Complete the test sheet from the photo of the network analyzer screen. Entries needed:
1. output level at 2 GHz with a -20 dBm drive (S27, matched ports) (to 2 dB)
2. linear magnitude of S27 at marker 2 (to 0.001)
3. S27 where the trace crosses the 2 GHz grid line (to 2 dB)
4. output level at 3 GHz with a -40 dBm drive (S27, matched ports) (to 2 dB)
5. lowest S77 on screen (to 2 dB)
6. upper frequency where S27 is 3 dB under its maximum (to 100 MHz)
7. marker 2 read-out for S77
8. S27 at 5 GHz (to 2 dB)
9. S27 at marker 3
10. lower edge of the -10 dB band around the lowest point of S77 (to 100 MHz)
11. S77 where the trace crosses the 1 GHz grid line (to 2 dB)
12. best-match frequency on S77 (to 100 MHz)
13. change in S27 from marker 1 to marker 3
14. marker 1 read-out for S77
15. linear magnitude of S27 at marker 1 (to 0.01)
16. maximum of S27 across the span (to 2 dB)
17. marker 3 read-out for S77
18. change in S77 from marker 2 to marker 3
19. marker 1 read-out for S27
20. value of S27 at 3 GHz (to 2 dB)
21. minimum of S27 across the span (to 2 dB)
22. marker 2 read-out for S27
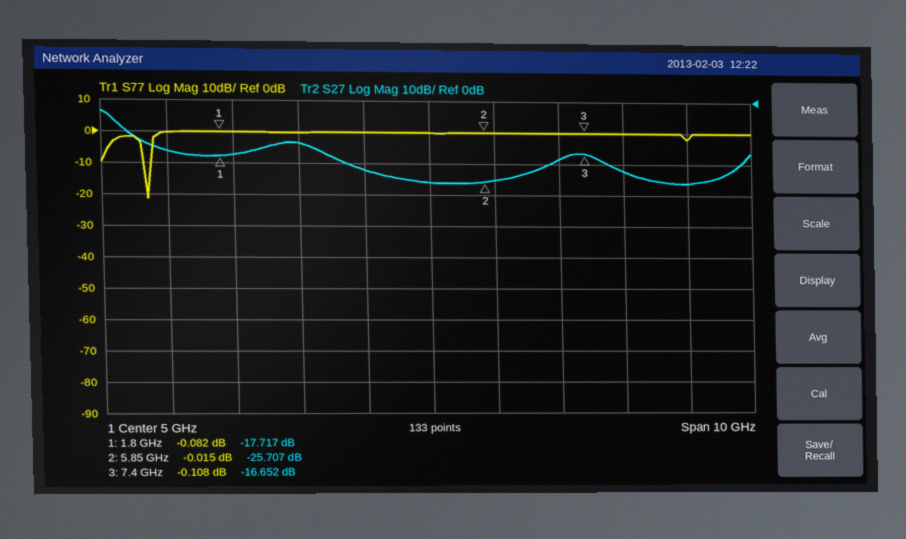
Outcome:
-38 dBm
0.052
-18 dB
-54 dBm
-22 dB
200 MHz
-0.015 dB
-26 dB
-16.652 dB
600 MHz
0 dB
700 MHz
1.065 dB
-0.082 dB
0.13
-4 dB
-0.108 dB
-0.093 dB
-17.717 dB
-14 dB
-26 dB
-25.707 dB
